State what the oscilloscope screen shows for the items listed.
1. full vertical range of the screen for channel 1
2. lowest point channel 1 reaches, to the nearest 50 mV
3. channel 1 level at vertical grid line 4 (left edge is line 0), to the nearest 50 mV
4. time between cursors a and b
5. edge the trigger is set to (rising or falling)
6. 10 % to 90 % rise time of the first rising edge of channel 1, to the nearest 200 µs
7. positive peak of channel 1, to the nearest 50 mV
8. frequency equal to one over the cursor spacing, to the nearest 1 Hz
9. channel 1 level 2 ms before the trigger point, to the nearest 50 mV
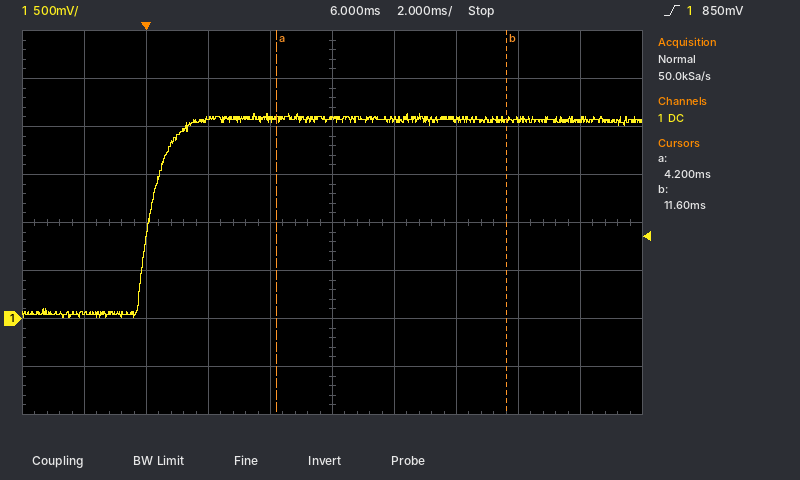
4 V
0 mV
2.10 V
7.4 ms
rising
1.2 ms
2.15 V
135 Hz
50 mV
